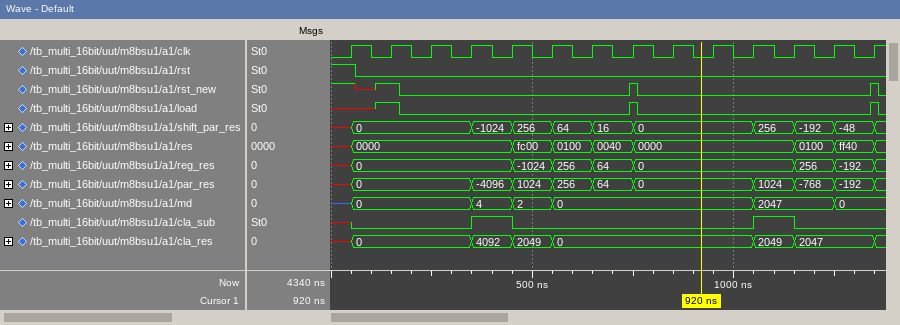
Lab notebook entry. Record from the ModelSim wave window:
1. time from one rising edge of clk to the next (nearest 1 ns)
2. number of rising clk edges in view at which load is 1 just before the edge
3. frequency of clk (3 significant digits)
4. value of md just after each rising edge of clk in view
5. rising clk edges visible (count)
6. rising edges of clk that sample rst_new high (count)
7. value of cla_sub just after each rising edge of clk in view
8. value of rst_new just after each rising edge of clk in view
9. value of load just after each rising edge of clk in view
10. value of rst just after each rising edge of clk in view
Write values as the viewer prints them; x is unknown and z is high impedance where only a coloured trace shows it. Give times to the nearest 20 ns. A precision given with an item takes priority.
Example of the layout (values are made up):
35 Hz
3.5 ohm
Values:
100 ns
3
10.0 MHz
0, 0, 0, 4, 2, 0, 0, 0, 0, 0, 2047, 2047, 0, 0
14
4
0 0 0 1 0 0 0 0 0 0 1 0 0 0
1 1 0 0 0 0 0 1 0 0 0 0 0 1
x 1 0 0 0 0 0 1 0 0 0 0 0 1
1 0 0 0 0 0 0 0 0 0 0 0 0 0
